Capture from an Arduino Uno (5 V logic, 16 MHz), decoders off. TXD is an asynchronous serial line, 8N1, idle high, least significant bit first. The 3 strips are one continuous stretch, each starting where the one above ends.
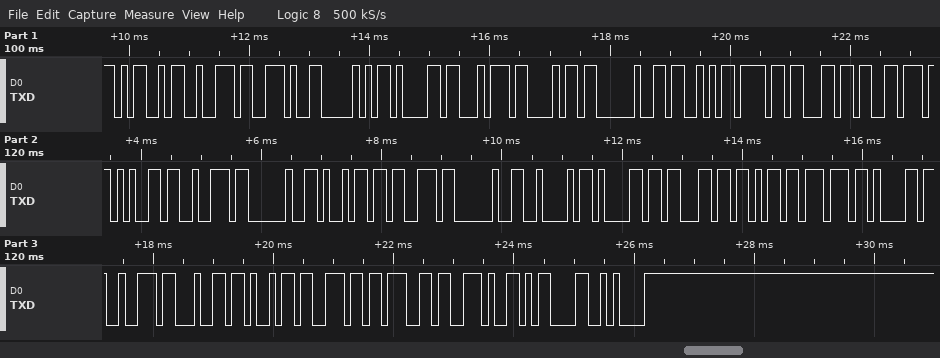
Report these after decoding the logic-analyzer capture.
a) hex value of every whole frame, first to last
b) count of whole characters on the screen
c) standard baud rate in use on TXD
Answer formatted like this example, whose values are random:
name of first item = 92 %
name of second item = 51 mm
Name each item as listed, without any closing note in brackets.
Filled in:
hex value of every whole frame, first to last = 4D 72 2E 50 61 74 68 20 53 6F 6C 76 65 72 20 69 73 20 42 61 63 6B 77 61 72 64 69 6E 67 2E 0D 0A
count of whole characters on the screen = 32
standard baud rate in use on TXD = 9600 baud
